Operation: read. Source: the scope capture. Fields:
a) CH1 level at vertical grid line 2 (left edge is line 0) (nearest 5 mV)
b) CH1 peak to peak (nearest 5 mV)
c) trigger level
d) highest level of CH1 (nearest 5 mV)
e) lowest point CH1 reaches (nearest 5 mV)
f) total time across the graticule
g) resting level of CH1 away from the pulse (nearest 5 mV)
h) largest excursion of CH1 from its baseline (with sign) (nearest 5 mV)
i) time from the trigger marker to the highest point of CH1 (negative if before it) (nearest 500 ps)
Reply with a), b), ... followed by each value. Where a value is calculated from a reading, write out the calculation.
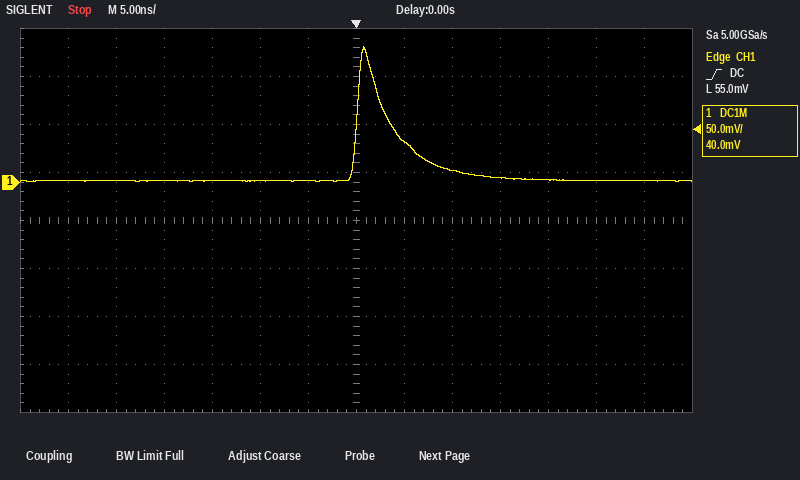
a) 0 mV
b) 140 mV − (0 mV) = 140 mV
c) 55.0 mV
d) 140 mV
e) 0 mV
f) 70 ns
g) 0 mV
h) 140 mV − (0 mV) = +140 mV
i) +1.0 ns
